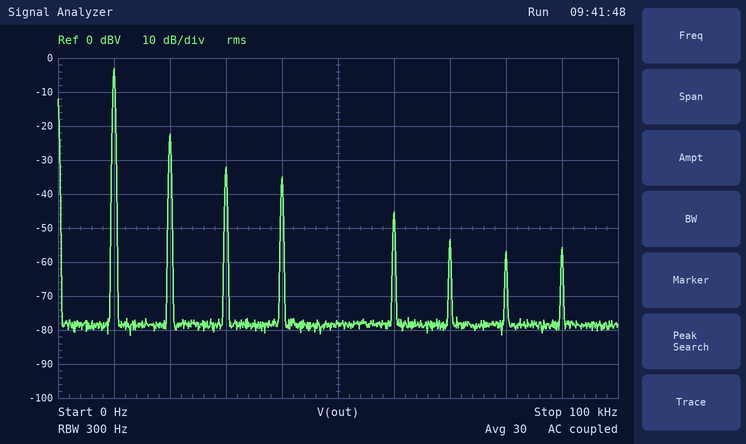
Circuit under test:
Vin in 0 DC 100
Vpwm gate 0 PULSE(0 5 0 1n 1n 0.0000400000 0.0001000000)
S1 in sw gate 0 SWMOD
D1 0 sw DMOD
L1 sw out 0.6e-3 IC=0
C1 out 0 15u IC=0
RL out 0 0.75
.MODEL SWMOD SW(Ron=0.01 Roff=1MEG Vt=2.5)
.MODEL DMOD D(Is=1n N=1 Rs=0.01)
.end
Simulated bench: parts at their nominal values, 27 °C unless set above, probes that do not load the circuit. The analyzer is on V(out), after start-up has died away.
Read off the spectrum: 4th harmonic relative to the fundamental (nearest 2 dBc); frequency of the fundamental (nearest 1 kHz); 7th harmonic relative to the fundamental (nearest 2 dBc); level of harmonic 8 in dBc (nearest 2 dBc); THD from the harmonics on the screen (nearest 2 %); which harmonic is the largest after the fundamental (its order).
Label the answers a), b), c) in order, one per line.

a) -32 dBc
b) 10 kHz
c) -50 dBc
d) -54 dBc
e) 12 %
f) 2
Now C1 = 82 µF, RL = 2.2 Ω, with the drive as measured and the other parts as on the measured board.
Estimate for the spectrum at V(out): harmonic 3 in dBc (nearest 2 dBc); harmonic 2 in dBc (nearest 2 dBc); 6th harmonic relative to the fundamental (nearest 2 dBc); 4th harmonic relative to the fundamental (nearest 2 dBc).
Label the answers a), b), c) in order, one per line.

a) -32 dBc
b) -22 dBc
c) -46 dBc
d) -36 dBc
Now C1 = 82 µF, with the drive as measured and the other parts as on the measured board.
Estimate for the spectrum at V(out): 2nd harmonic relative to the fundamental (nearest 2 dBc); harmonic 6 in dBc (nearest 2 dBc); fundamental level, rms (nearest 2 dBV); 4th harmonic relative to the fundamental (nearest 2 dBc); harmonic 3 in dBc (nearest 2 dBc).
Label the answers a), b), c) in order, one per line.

a) -22 dBc
b) -46 dBc
c) -14 dBV
d) -36 dBc
e) -32 dBc
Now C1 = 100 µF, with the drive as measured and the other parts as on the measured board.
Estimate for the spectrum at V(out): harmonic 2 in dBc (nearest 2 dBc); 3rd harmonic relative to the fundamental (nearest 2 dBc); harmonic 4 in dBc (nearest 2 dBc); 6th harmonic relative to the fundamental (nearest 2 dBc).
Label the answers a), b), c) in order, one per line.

a) -22 dBc
b) -32 dBc
c) -36 dBc
d) -46 dBc
